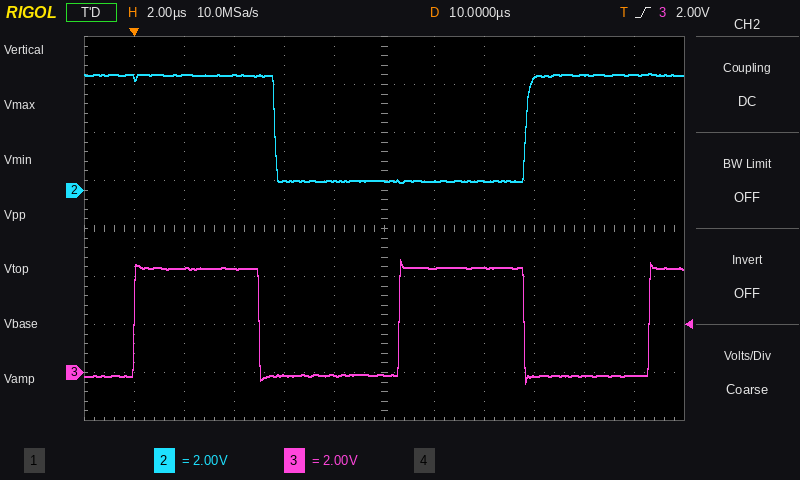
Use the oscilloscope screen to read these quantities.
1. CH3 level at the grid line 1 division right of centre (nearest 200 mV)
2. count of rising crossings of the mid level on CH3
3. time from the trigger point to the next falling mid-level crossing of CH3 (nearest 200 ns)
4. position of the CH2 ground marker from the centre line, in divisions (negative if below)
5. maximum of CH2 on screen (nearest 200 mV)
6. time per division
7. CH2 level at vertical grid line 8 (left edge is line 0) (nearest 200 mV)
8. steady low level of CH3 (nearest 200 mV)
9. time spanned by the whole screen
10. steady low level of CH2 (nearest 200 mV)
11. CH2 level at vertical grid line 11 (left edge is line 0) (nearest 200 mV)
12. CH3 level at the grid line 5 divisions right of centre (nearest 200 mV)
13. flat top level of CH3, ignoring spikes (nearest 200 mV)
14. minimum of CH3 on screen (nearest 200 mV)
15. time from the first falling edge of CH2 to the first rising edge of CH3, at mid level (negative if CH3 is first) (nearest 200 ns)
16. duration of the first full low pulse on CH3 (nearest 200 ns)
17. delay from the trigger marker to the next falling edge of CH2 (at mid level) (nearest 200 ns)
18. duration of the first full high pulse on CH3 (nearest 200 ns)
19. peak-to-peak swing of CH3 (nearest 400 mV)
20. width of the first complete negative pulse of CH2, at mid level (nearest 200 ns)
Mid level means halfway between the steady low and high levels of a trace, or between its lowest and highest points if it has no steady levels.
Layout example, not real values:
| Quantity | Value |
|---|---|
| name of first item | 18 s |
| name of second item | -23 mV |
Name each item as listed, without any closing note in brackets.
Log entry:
| Quantity | Value |
|---|---|
| CH3 level at the grid line 1 division right of centre | 4.4 V |
| count of rising crossings of the mid level on CH3 | 3 |
| time from the trigger point to the next falling mid-level crossing of CH3 | 5.0 µs |
| position of the CH2 ground marker from the centre line, in divisions | +0.8 div |
| maximum of CH2 on screen | 4.8 V |
| time per division | 2 µs |
| CH2 level at vertical grid line 8 (left edge is line 0) | 400 mV |
| steady low level of CH3 | -200 mV |
| time spanned by the whole screen | 24 µs |
| steady low level of CH2 | 400 mV |
| CH2 level at vertical grid line 11 (left edge is line 0) | 4.8 V |
| CH3 level at the grid line 5 divisions right of centre | -200 mV |
| flat top level of CH3, ignoring spikes | 4.4 V |
| minimum of CH3 on screen | -400 mV |
| time from the first falling edge of CH2 to the first rising edge of CH3, at mid level (negative if CH3 is first) | -5.6 µs |
| duration of the first full low pulse on CH3 | 5.6 µs |
| delay from the trigger marker to the next falling edge of CH2 (at mid level) | 5.6 µs |
| duration of the first full high pulse on CH3 | 5.0 µs |
| peak-to-peak swing of CH3 | 5.2 V |
| width of the first complete negative pulse of CH2, at mid level | 10.0 µs |
